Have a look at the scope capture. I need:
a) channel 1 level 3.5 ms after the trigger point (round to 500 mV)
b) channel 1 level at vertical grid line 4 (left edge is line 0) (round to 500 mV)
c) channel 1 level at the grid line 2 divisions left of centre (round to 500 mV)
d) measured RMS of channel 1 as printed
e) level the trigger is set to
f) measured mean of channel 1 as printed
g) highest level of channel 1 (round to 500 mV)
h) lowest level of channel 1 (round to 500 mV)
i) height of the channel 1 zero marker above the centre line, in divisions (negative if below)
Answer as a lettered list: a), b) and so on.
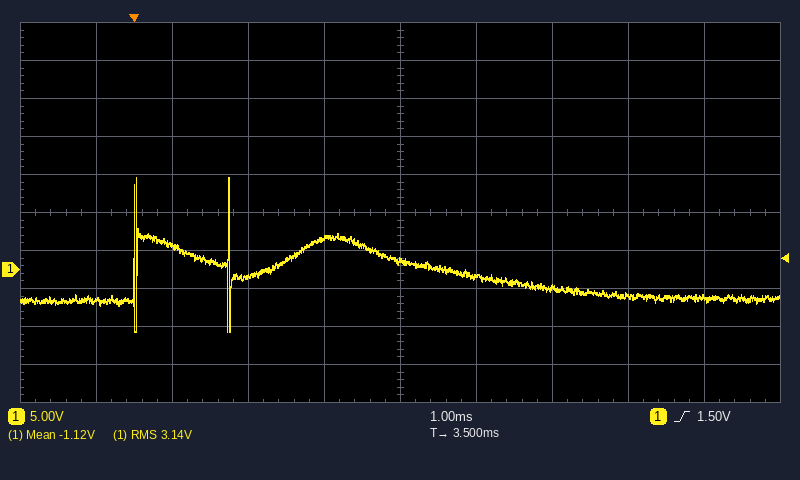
a) 1.0 V
b) 4.0 V
c) -1.0 V
d) 3.14 V
e) 1.50 V
f) -1.12 V
g) 12.0 V
h) -8.0 V
i) -1.5 div
